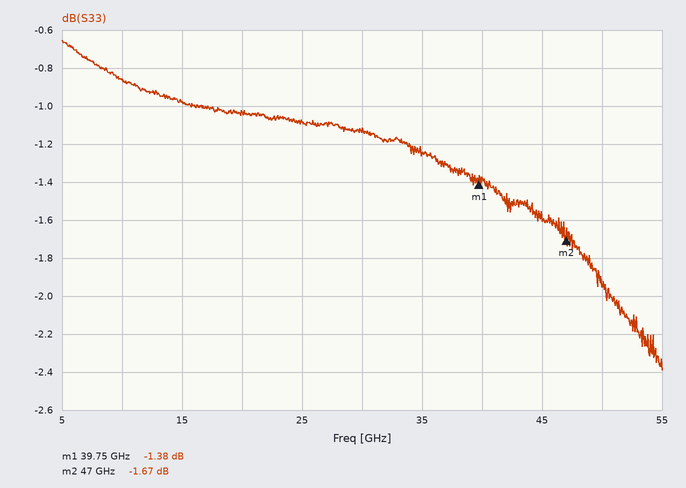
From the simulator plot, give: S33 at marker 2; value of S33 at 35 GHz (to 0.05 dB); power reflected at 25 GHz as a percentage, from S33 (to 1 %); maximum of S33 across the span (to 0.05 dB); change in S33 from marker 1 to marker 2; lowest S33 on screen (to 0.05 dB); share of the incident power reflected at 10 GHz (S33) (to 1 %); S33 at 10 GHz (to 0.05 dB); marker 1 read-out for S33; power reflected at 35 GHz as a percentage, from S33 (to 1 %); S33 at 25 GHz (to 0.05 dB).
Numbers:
-1.67 dB
-1.25 dB
78 %
-0.65 dB
-0.29 dB
-2.40 dB
82 %
-0.85 dB
-1.38 dB
75 %
-1.10 dB
